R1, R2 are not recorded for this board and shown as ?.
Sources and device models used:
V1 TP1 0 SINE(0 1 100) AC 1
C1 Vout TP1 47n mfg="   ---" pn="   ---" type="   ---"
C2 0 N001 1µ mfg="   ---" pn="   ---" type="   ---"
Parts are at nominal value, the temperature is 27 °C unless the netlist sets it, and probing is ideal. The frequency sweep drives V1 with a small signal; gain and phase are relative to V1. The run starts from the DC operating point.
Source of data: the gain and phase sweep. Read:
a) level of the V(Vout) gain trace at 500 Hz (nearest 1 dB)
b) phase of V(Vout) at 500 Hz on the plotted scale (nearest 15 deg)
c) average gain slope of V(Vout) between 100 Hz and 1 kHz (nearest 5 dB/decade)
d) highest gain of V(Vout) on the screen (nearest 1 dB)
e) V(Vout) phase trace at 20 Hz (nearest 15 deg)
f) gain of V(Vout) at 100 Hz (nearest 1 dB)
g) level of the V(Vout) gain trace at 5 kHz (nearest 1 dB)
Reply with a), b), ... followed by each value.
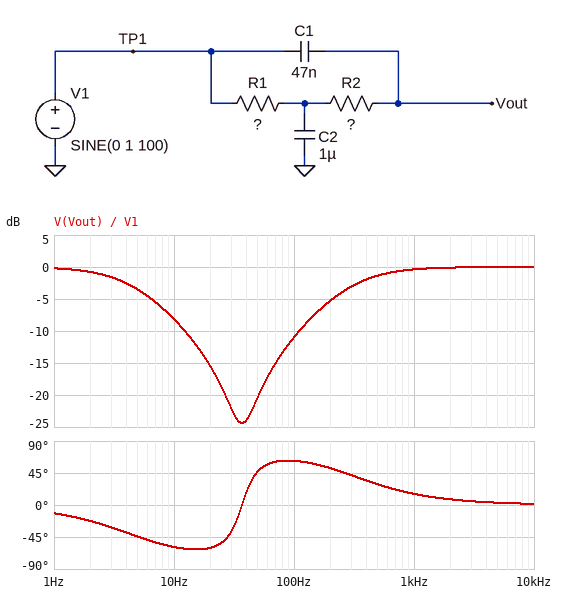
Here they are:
a) -1 dB
b) 30 deg
c) 10 dB/decade
d) 0 dB
e) -60 deg
f) -11 dB
g) 0 dB
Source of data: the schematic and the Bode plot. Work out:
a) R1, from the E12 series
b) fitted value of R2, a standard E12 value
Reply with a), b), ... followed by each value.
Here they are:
a) 33 kΩ
b) 12 kΩ
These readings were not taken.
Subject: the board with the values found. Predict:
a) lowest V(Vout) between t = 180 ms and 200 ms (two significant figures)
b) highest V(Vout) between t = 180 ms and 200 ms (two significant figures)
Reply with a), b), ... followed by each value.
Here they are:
a) -280 mV
b) 280 mV
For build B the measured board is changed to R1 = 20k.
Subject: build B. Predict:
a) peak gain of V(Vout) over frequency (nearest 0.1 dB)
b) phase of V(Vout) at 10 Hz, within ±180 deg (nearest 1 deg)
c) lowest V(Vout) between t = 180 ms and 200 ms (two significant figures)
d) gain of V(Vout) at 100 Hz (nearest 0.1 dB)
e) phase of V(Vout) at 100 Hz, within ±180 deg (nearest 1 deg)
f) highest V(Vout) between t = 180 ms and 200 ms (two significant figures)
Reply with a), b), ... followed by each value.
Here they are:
a) 0 dB
b) -49 deg
c) -260 mV
d) -11.8 dB
e) 60 deg
f) 260 mV
